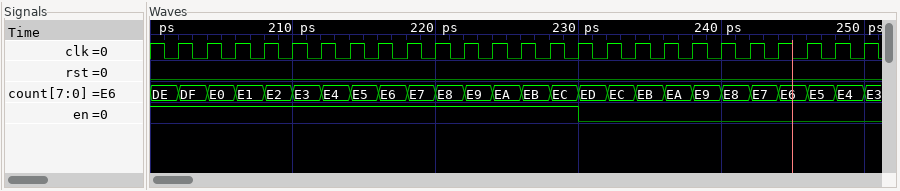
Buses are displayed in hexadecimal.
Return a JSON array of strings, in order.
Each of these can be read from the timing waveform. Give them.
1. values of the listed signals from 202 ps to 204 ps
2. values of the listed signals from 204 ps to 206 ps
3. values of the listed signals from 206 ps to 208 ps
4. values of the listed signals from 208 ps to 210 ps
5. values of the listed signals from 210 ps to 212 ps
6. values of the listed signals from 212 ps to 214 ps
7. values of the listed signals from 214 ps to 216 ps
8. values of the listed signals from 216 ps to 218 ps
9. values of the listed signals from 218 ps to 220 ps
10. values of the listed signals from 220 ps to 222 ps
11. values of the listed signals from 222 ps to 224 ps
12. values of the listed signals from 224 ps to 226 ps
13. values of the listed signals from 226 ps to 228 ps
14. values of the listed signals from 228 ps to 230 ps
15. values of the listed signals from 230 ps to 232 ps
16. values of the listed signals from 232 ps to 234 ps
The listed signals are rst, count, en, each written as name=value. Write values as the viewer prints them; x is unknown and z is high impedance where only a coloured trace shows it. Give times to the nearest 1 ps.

["rst=0, count=DF, en=1", "rst=0, count=E0, en=1", "rst=0, count=E1, en=1", "rst=0, count=E2, en=1", "rst=0, count=E3, en=1", "rst=0, count=E4, en=1", "rst=0, count=E5, en=1", "rst=0, count=E6, en=1", "rst=0, count=E7, en=1", "rst=0, count=E8, en=1", "rst=0, count=E9, en=1", "rst=0, count=EA, en=1", "rst=0, count=EB, en=1", "rst=0, count=EC, en=1", "rst=0, count=ED, en=0", "rst=0, count=EC, en=0"]
